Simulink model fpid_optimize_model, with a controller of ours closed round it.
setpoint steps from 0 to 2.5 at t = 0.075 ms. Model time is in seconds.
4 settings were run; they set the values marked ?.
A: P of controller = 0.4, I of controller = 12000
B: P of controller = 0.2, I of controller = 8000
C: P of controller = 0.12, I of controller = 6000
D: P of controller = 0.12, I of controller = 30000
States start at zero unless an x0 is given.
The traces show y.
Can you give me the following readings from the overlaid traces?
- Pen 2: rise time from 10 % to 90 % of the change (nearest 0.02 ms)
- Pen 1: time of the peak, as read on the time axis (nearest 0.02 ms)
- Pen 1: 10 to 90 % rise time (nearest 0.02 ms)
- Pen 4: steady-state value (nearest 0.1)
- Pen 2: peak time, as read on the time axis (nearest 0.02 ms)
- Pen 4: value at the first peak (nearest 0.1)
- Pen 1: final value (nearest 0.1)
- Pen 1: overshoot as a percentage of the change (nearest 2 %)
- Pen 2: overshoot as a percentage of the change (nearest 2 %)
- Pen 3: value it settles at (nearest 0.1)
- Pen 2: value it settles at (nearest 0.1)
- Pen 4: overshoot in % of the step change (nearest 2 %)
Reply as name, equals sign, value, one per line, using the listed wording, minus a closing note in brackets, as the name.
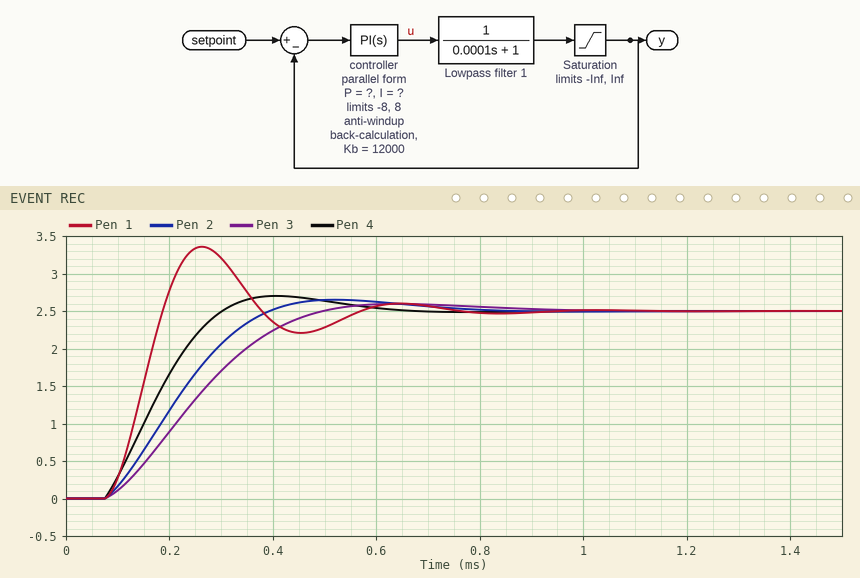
Pen 2: rise time from 10 % to 90 % of the change = 0.22 ms
Pen 1: time of the peak, as read on the time axis = 0.26 ms
Pen 1: 10 to 90 % rise time = 0.08 ms
Pen 4: steady-state value = 2.5
Pen 2: peak time, as read on the time axis = 0.52 ms
Pen 4: value at the first peak = 2.7
Pen 1: final value = 2.5
Pen 1: overshoot as a percentage of the change = 34 %
Pen 2: overshoot as a percentage of the change = 6 %
Pen 3: value it settles at = 2.5
Pen 2: value it settles at = 2.5
Pen 4: overshoot in % of the step change = 8 %
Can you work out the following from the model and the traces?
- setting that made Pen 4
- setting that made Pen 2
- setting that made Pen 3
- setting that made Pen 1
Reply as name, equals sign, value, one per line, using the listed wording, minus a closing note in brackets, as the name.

setting that made Pen 4 = A
setting that made Pen 2 = B
setting that made Pen 3 = C
setting that made Pen 1 = D
